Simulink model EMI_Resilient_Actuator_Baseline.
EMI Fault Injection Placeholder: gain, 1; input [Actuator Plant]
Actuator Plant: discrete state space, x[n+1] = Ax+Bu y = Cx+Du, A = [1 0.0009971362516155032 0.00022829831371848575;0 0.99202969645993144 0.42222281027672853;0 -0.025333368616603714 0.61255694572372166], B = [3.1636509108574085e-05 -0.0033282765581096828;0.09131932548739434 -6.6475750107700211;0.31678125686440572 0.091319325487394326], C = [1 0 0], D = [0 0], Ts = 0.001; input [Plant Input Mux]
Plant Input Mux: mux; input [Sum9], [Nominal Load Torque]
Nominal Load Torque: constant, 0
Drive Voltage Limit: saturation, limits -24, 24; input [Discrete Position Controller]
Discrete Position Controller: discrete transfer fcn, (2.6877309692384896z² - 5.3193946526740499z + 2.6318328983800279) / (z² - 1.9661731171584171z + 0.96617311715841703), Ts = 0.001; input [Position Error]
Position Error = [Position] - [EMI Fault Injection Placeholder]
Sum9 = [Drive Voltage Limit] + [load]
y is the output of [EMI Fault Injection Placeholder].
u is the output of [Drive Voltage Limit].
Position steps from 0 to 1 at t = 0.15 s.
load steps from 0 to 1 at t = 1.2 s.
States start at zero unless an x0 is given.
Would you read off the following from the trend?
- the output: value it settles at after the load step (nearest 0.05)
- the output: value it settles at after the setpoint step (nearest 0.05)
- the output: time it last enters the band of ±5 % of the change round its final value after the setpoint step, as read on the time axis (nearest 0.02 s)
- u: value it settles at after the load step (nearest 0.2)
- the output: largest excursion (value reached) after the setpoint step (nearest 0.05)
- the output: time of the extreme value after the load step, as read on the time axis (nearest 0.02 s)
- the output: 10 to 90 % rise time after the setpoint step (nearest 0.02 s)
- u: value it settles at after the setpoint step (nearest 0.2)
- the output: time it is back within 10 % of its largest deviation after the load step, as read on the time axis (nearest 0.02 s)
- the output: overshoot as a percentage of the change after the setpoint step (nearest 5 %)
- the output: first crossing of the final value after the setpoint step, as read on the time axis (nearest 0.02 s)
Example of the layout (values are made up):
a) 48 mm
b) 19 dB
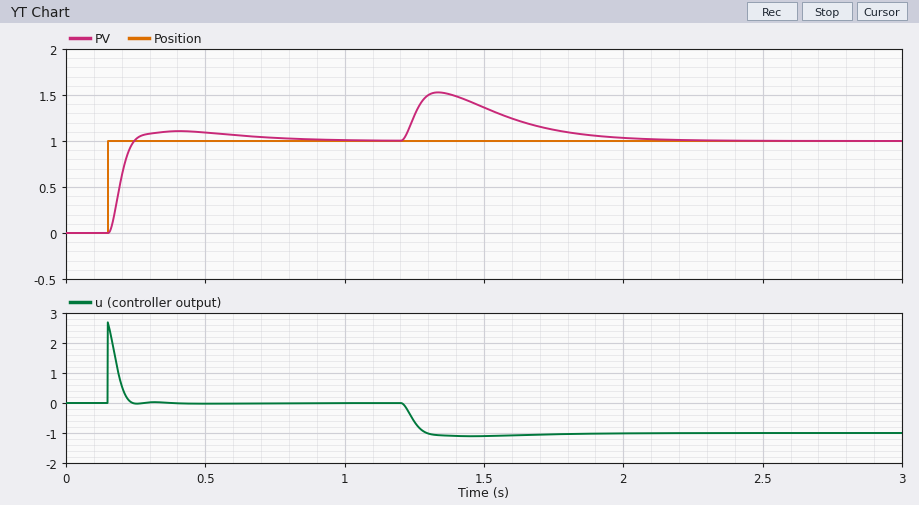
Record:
a) 1.00
b) 1.00
c) 0.66 s
d) -1.0
e) 1.10
f) 1.34 s
g) 0.06 s
h) 0.0
i) 1.92 s
j) 10 %
k) 0.24 s
